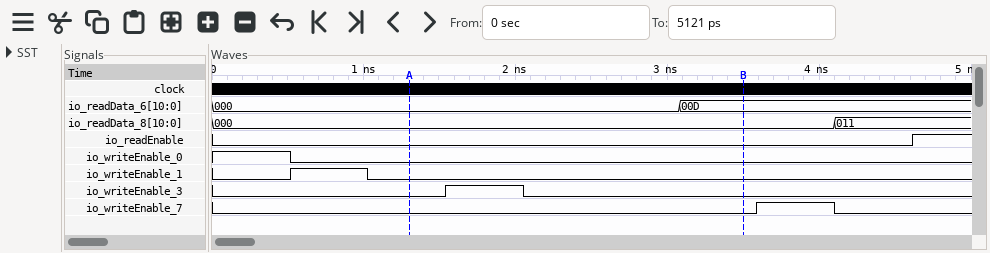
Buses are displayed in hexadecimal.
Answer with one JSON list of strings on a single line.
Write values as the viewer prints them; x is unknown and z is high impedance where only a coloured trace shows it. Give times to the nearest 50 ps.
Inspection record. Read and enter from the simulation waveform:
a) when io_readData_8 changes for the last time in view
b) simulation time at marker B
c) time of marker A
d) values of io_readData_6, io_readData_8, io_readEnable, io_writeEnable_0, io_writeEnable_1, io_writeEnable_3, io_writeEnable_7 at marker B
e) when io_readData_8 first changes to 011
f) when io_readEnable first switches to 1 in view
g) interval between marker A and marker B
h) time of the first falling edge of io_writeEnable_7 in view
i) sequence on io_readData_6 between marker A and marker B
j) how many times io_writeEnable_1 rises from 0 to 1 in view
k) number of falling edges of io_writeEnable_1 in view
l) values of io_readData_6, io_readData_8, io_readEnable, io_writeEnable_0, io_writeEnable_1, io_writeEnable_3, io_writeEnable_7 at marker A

["4100 ps", "3500 ps", "1300 ps", "io_readData_6=00D, io_readData_8=000, io_readEnable=0, io_writeEnable_0=0, io_writeEnable_1=0, io_writeEnable_3=0, io_writeEnable_7=0", "4100 ps", "4600 ps", "2200 ps", "4100 ps", "000, 00D", "1", "1", "io_readData_6=000, io_readData_8=000, io_readEnable=0, io_writeEnable_0=0, io_writeEnable_1=0, io_writeEnable_3=0, io_writeEnable_7=0"]
